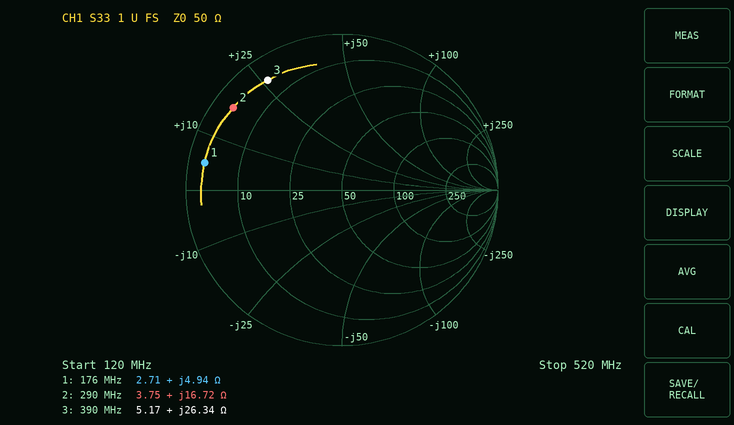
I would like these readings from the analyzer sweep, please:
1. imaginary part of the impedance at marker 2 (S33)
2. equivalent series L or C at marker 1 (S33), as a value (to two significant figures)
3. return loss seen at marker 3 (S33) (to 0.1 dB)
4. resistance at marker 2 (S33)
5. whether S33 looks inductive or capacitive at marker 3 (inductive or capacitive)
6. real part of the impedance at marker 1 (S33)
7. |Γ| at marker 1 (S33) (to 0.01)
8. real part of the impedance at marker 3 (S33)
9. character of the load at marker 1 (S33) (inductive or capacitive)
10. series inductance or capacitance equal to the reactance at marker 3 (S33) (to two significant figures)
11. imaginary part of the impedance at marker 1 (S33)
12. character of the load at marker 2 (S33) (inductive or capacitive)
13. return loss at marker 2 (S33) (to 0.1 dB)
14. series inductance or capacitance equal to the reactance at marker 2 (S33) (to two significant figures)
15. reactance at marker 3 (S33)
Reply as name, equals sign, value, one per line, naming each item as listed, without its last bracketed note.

imaginary part of the impedance at marker 2 = +16.72 Ω
equivalent series L or C at marker 1 (S33), as a value = 4.5 nH
return loss seen at marker 3 (S33) = 1.4 dB
resistance at marker 2 = 3.75 Ω
whether S33 looks inductive or capacitive at marker 3 = inductive
real part of the impedance at marker 1 = 2.71 Ω
|Γ| at marker 1 (S33) = 0.90
real part of the impedance at marker 3 = 5.17 Ω
character of the load at marker 1 (S33) = inductive
series inductance or capacitance equal to the reactance at marker 3 (S33) = 11 nH
imaginary part of the impedance at marker 1 = +4.94 Ω
character of the load at marker 2 (S33) = inductive
return loss at marker 2 (S33) = 1.2 dB
series inductance or capacitance equal to the reactance at marker 2 (S33) = 9.2 nH
reactance at marker 3 = +26.34 Ω
